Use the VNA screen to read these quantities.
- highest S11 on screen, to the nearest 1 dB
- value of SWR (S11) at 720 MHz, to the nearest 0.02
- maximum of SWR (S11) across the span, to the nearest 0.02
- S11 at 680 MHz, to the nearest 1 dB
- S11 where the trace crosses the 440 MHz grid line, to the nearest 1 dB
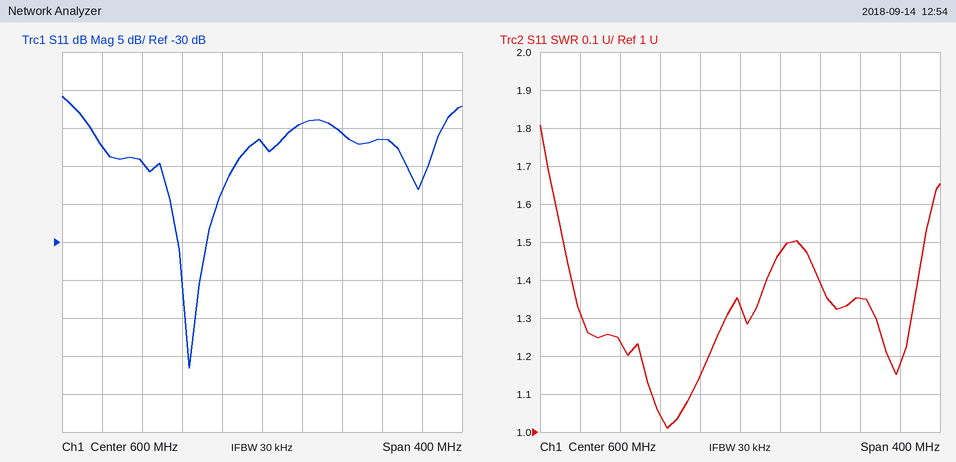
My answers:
-11 dB
1.36
1.80
-16 dB
-17 dB
